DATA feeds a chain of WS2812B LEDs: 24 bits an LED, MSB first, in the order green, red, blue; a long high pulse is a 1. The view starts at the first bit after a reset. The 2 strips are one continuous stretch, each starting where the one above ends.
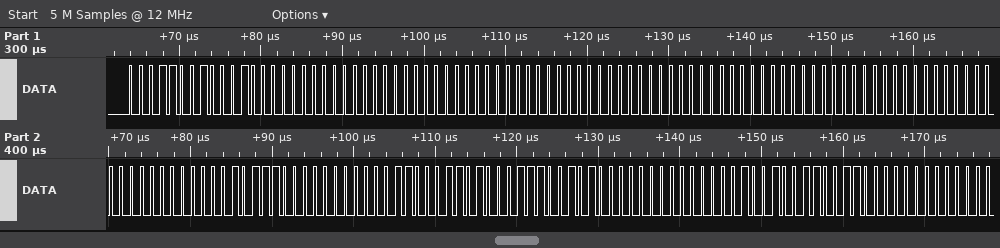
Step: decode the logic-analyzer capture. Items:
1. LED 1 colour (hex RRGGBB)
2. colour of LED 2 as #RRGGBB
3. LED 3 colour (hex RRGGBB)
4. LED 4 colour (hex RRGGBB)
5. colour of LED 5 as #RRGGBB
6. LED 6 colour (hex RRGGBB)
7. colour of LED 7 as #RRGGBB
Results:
#101900
#000000
#000000
#000000
#005C63
#284700
#661200
